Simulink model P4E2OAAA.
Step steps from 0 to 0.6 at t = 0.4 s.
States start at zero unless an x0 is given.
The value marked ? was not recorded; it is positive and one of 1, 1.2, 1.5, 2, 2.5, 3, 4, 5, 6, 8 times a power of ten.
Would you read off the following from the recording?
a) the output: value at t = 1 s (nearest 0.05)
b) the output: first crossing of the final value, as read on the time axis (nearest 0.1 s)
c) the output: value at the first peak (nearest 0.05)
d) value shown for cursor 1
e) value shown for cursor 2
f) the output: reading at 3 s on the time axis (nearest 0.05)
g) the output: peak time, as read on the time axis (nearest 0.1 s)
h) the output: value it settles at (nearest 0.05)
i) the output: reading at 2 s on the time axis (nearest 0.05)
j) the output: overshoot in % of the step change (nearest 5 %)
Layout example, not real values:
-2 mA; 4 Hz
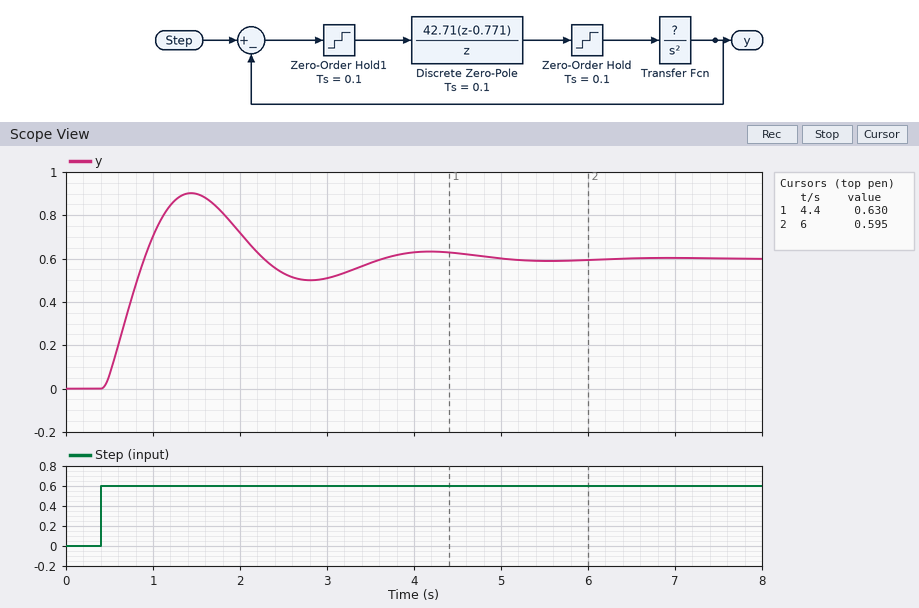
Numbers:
0.70; 0.9 s; 0.90; 0.630; 0.595; 0.50; 1.4 s; 0.60; 0.70; 50 %
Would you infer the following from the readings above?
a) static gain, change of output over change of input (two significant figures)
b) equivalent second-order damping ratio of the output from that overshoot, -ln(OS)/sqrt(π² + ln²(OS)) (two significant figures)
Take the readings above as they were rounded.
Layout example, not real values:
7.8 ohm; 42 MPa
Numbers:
1.0; 0.22
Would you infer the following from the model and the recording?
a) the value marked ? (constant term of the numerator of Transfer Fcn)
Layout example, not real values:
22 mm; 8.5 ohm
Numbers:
0.5
